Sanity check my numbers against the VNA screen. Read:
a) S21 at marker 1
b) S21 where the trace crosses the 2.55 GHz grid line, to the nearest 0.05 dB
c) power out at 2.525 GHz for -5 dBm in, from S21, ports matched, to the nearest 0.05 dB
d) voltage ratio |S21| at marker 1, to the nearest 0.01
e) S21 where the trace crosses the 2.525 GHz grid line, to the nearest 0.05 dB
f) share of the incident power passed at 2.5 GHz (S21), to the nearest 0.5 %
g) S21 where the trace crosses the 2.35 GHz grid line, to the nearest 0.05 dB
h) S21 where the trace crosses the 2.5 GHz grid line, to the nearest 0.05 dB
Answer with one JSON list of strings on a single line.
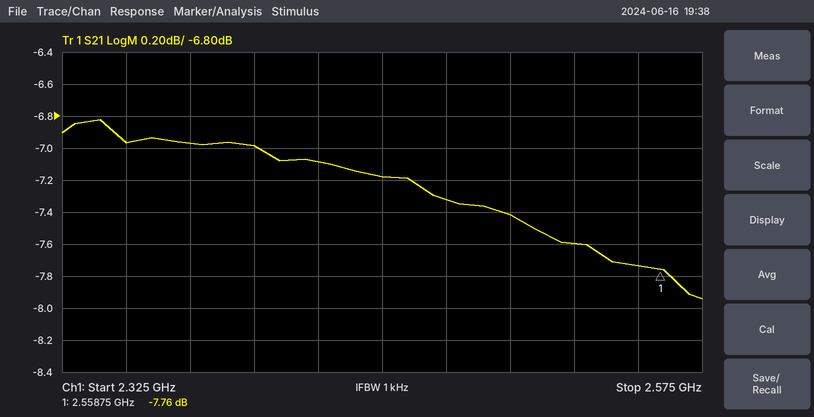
["-7.76 dB", "-7.75 dB", "-12.60 dBm", "0.41", "-7.60 dB", "18.0 %", "-6.95 dB", "-7.40 dB"]
